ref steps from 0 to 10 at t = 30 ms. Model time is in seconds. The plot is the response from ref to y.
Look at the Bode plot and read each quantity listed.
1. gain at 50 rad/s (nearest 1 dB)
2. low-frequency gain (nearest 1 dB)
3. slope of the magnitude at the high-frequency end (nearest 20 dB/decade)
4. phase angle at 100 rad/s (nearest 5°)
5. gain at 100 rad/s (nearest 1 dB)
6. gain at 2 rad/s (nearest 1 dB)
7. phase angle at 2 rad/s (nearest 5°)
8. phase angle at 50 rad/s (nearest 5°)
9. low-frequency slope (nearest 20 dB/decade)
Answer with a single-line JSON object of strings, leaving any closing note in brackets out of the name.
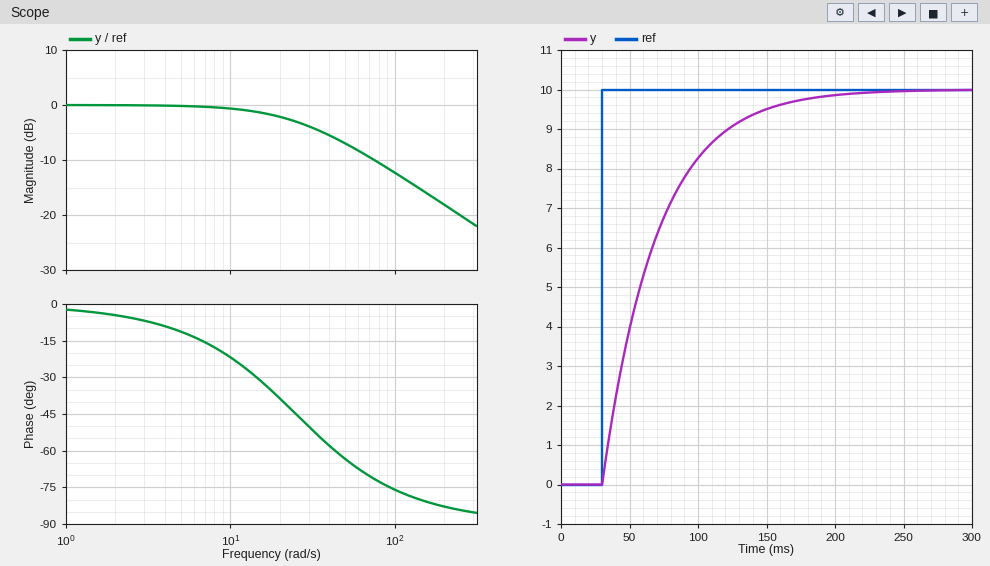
{"gain at 50 rad/s": "-7 dB", "low-frequency gain": "0 dB", "slope of the magnitude at the high-frequency end": "-20 dB/decade", "phase angle at 100 rad/s": "-75°", "gain at 100 rad/s": "-12 dB", "gain at 2 rad/s": "0 dB", "phase angle at 2 rad/s": "-5°", "phase angle at 50 rad/s": "-65°", "low-frequency slope": "0 dB/decade"}
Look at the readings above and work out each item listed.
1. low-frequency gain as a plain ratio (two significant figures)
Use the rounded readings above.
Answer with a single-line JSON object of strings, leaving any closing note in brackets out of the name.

{"low-frequency gain as a plain ratio": "1.0"}
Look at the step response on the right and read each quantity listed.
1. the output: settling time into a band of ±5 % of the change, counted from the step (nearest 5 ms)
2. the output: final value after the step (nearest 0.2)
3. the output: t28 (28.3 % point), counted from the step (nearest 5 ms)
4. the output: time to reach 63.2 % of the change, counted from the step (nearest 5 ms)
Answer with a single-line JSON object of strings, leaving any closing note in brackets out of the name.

{"the output: settling time into a band of ±5 % of the change, counted from the step": "120 ms", "the output: final value after the step": "10.0", "the output: t28 (28.3 % point), counted from the step": "15 ms", "the output: time to reach 63.2 % of the change, counted from the step": "40 ms"}
